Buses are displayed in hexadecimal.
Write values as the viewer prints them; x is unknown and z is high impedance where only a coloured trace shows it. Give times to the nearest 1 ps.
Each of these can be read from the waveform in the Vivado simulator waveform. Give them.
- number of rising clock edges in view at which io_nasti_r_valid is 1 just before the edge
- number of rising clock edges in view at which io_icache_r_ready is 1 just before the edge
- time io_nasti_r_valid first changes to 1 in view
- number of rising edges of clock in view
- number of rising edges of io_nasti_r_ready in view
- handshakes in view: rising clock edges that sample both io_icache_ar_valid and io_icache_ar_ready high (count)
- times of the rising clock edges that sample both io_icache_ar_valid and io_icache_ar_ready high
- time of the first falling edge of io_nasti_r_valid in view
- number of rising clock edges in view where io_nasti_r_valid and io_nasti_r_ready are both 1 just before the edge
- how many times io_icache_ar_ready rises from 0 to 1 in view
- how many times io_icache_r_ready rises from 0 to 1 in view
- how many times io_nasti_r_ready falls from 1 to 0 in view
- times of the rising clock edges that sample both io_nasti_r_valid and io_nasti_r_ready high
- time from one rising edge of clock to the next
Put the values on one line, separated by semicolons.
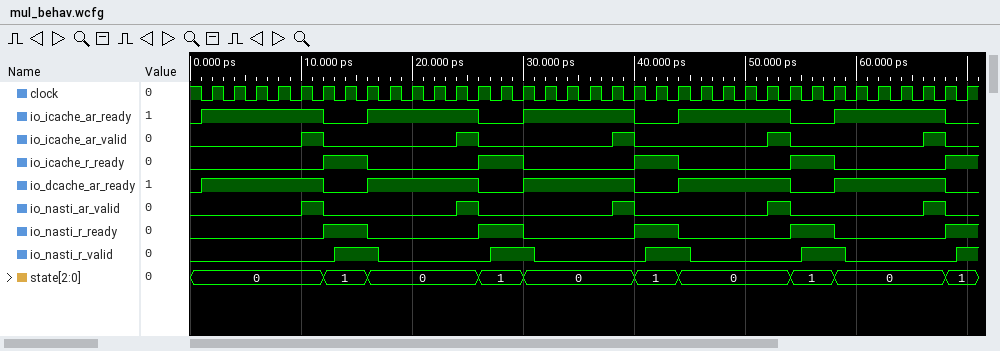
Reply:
9; 9; 13 ps; 35; 5; 5; 12 ps, 26 ps, 40 ps, 54 ps, 68 ps; 17 ps; 9; 5; 5; 4; 14 ps, 16 ps, 28 ps, 30 ps, 42 ps, 44 ps, 56 ps, 58 ps, 70 ps; 2 ps
